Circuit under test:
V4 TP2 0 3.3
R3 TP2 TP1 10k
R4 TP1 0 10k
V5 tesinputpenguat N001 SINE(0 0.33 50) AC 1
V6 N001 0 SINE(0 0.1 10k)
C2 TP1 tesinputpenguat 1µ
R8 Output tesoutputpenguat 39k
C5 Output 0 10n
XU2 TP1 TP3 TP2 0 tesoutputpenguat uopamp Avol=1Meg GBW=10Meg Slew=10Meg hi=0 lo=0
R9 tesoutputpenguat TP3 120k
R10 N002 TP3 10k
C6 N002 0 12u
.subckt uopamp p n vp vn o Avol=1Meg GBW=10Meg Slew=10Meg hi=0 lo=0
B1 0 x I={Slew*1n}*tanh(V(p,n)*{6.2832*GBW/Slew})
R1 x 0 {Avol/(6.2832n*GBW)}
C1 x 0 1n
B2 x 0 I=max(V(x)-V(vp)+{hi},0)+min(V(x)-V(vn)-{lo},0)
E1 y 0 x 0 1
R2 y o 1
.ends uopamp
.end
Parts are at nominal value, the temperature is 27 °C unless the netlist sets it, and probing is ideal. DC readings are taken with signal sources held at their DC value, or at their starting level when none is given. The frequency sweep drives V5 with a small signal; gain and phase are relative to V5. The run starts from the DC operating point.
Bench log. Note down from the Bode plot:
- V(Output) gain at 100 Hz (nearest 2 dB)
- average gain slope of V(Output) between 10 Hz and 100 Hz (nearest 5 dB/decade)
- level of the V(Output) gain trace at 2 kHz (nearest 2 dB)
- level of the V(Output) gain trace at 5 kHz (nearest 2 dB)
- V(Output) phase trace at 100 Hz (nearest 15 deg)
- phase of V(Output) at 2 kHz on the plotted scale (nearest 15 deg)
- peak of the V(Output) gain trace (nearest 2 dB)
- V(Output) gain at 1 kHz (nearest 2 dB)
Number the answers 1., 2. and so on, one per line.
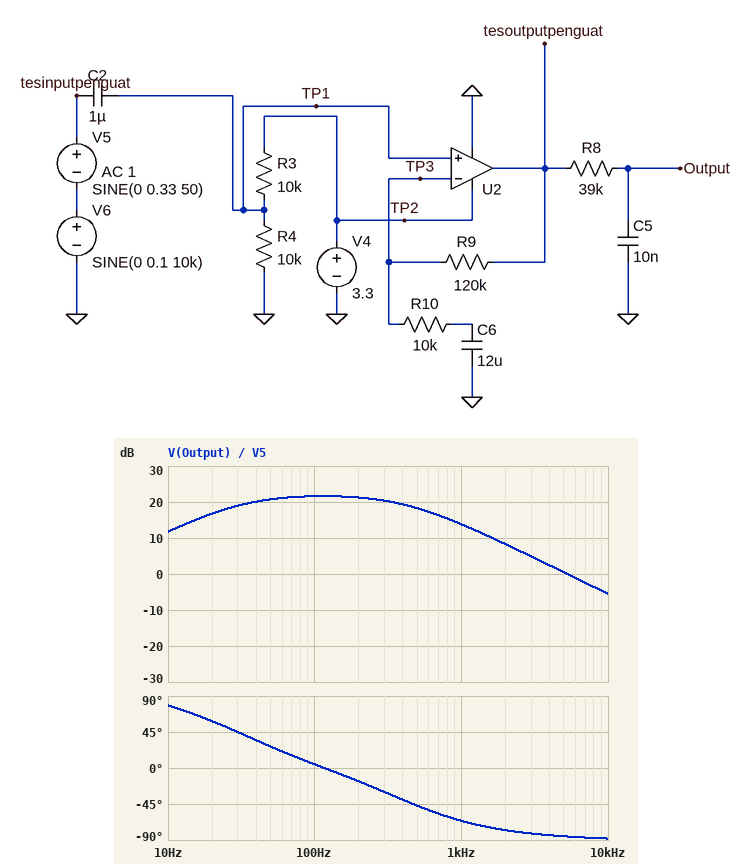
1. 22 dB
2. 10 dB/decade
3. 8 dB
4. 0 dB
5. 0 deg
6. -75 deg
7. 22 dB
8. 14 dB
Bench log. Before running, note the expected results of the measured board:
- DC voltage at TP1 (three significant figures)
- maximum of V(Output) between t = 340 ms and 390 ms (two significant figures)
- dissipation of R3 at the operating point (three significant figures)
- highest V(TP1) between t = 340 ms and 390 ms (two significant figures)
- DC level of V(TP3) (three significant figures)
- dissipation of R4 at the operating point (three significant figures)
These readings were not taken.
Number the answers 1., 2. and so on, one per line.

1. 1.65 V
2. 3.3 V
3. 272 µW
4. 2.0 V
5. 1.65 V
6. 272 µW
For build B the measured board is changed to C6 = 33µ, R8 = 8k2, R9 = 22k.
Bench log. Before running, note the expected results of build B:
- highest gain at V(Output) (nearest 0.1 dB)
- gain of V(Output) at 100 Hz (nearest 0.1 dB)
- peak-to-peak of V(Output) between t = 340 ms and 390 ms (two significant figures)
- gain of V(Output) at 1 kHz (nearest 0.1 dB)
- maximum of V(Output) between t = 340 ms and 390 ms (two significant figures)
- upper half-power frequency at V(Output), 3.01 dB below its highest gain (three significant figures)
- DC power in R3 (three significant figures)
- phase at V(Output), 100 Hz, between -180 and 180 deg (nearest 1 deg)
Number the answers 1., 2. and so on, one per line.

1. 10.0 dB
2. 9.7 dB
3. 1.9 V
4. 9.1 dB
5. 2.6 V
6. 2.00 kHz
7. 272 µW
8. 15 deg
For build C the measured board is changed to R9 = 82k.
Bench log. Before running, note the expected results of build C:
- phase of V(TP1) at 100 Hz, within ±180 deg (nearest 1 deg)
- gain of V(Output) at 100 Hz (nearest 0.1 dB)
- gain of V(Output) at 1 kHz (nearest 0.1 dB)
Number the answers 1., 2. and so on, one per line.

1. 18 deg
2. 18.6 dB
3. 10.8 dB
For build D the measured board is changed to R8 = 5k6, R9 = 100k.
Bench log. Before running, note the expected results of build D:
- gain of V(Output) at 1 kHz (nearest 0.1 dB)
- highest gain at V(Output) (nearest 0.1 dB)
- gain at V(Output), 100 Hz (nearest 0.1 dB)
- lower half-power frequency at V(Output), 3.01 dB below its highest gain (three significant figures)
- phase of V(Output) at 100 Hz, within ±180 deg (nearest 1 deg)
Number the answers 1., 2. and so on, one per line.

1. 20.3 dB
2. 20.7 dB
3. 20.4 dB
4. 31.2 Hz
5. 16 deg
